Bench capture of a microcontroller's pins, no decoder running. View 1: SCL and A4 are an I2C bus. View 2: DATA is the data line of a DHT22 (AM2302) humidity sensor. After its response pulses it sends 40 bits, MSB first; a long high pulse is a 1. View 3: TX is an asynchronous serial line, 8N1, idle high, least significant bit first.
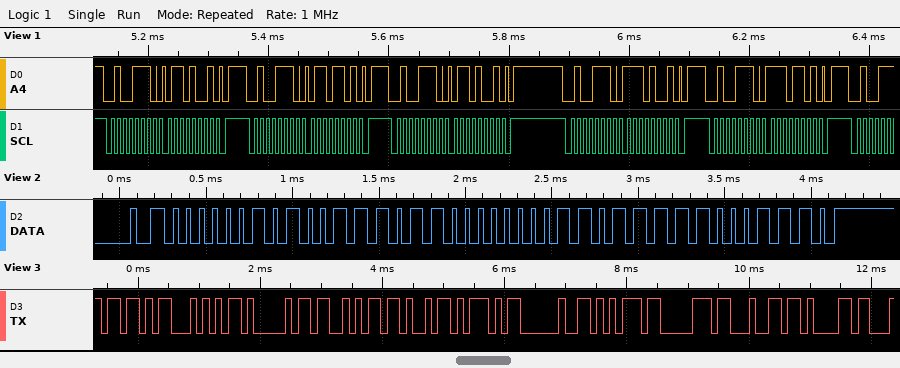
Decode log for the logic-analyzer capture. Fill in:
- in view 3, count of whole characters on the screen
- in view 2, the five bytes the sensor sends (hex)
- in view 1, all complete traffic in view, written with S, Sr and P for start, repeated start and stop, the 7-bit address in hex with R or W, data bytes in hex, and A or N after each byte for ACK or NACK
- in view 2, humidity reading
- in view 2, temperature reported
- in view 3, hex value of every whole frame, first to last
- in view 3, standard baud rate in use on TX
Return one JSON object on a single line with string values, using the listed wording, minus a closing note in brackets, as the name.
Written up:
{"in view 3, count of whole characters on the screen": "11", "in view 2, the five bytes the sensor sends": "02 9D 80 6F 8E", "in view 1, all complete traffic in view, written with S, Sr and P for start, repeated start and stop, the 7-bit address in hex with R or W, data bytes in hex, and A or N after each byte for ACK or NACK": "S 27W A 69 A P S 27W A 6D A P S 27W A 69 A P S 27W A E9 A P S 27W A ED A P", "in view 2, humidity reading": "66.9 %", "in view 2, temperature reported": "-11.1 °C", "in view 3, hex value of every whole frame, first to last": "0x5B 0x54 0x41 0x53 0x4B 0x5D 0x20 0x75 0x70 0x64 0x61", "in view 3, standard baud rate in use on TX": "9600 baud"}
